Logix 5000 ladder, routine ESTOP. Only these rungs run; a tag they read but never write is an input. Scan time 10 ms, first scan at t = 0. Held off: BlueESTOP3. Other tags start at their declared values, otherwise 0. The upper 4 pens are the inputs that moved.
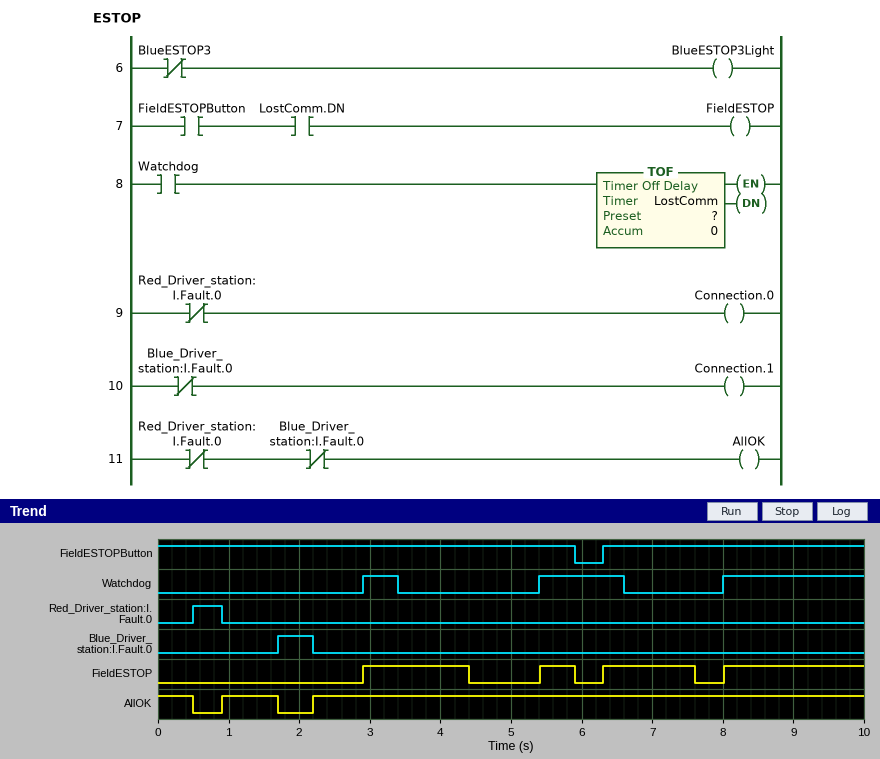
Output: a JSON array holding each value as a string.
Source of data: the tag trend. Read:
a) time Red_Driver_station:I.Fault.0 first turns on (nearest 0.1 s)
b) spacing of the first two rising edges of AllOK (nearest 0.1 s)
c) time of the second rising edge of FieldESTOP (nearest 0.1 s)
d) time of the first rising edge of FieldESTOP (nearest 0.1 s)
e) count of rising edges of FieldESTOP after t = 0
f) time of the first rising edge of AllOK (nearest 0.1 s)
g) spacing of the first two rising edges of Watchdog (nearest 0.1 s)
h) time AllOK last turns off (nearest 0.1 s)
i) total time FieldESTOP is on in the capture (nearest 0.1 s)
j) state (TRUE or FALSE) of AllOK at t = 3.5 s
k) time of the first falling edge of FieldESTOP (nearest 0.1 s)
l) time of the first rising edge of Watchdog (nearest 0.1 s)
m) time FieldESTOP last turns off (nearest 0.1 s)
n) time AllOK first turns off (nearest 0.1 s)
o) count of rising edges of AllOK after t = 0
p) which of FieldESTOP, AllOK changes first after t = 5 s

["0.5 s", "1.3 s", "5.4 s", "2.9 s", "4", "0.9 s", "2.5 s", "1.7 s", "5.3 s", "TRUE", "4.4 s", "2.9 s", "7.6 s", "0.5 s", "2", "FieldESTOP"]
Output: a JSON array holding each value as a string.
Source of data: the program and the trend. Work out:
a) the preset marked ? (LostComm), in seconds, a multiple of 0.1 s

["1.0 s"]
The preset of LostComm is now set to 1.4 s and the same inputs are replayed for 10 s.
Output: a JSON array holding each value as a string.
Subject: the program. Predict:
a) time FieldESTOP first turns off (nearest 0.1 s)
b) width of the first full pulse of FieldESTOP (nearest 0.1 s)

["4.8 s", "1.9 s"]
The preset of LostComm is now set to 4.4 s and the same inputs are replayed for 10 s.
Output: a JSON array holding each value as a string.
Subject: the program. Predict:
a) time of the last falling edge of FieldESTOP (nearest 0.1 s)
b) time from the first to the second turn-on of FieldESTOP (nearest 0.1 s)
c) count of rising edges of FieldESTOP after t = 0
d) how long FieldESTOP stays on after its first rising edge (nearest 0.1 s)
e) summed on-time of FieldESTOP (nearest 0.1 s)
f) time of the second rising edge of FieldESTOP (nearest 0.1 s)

["5.9 s", "3.4 s", "2", "3.0 s", "6.7 s", "6.3 s"]
